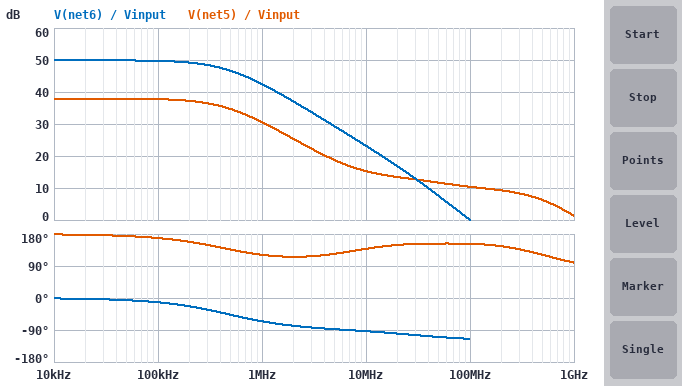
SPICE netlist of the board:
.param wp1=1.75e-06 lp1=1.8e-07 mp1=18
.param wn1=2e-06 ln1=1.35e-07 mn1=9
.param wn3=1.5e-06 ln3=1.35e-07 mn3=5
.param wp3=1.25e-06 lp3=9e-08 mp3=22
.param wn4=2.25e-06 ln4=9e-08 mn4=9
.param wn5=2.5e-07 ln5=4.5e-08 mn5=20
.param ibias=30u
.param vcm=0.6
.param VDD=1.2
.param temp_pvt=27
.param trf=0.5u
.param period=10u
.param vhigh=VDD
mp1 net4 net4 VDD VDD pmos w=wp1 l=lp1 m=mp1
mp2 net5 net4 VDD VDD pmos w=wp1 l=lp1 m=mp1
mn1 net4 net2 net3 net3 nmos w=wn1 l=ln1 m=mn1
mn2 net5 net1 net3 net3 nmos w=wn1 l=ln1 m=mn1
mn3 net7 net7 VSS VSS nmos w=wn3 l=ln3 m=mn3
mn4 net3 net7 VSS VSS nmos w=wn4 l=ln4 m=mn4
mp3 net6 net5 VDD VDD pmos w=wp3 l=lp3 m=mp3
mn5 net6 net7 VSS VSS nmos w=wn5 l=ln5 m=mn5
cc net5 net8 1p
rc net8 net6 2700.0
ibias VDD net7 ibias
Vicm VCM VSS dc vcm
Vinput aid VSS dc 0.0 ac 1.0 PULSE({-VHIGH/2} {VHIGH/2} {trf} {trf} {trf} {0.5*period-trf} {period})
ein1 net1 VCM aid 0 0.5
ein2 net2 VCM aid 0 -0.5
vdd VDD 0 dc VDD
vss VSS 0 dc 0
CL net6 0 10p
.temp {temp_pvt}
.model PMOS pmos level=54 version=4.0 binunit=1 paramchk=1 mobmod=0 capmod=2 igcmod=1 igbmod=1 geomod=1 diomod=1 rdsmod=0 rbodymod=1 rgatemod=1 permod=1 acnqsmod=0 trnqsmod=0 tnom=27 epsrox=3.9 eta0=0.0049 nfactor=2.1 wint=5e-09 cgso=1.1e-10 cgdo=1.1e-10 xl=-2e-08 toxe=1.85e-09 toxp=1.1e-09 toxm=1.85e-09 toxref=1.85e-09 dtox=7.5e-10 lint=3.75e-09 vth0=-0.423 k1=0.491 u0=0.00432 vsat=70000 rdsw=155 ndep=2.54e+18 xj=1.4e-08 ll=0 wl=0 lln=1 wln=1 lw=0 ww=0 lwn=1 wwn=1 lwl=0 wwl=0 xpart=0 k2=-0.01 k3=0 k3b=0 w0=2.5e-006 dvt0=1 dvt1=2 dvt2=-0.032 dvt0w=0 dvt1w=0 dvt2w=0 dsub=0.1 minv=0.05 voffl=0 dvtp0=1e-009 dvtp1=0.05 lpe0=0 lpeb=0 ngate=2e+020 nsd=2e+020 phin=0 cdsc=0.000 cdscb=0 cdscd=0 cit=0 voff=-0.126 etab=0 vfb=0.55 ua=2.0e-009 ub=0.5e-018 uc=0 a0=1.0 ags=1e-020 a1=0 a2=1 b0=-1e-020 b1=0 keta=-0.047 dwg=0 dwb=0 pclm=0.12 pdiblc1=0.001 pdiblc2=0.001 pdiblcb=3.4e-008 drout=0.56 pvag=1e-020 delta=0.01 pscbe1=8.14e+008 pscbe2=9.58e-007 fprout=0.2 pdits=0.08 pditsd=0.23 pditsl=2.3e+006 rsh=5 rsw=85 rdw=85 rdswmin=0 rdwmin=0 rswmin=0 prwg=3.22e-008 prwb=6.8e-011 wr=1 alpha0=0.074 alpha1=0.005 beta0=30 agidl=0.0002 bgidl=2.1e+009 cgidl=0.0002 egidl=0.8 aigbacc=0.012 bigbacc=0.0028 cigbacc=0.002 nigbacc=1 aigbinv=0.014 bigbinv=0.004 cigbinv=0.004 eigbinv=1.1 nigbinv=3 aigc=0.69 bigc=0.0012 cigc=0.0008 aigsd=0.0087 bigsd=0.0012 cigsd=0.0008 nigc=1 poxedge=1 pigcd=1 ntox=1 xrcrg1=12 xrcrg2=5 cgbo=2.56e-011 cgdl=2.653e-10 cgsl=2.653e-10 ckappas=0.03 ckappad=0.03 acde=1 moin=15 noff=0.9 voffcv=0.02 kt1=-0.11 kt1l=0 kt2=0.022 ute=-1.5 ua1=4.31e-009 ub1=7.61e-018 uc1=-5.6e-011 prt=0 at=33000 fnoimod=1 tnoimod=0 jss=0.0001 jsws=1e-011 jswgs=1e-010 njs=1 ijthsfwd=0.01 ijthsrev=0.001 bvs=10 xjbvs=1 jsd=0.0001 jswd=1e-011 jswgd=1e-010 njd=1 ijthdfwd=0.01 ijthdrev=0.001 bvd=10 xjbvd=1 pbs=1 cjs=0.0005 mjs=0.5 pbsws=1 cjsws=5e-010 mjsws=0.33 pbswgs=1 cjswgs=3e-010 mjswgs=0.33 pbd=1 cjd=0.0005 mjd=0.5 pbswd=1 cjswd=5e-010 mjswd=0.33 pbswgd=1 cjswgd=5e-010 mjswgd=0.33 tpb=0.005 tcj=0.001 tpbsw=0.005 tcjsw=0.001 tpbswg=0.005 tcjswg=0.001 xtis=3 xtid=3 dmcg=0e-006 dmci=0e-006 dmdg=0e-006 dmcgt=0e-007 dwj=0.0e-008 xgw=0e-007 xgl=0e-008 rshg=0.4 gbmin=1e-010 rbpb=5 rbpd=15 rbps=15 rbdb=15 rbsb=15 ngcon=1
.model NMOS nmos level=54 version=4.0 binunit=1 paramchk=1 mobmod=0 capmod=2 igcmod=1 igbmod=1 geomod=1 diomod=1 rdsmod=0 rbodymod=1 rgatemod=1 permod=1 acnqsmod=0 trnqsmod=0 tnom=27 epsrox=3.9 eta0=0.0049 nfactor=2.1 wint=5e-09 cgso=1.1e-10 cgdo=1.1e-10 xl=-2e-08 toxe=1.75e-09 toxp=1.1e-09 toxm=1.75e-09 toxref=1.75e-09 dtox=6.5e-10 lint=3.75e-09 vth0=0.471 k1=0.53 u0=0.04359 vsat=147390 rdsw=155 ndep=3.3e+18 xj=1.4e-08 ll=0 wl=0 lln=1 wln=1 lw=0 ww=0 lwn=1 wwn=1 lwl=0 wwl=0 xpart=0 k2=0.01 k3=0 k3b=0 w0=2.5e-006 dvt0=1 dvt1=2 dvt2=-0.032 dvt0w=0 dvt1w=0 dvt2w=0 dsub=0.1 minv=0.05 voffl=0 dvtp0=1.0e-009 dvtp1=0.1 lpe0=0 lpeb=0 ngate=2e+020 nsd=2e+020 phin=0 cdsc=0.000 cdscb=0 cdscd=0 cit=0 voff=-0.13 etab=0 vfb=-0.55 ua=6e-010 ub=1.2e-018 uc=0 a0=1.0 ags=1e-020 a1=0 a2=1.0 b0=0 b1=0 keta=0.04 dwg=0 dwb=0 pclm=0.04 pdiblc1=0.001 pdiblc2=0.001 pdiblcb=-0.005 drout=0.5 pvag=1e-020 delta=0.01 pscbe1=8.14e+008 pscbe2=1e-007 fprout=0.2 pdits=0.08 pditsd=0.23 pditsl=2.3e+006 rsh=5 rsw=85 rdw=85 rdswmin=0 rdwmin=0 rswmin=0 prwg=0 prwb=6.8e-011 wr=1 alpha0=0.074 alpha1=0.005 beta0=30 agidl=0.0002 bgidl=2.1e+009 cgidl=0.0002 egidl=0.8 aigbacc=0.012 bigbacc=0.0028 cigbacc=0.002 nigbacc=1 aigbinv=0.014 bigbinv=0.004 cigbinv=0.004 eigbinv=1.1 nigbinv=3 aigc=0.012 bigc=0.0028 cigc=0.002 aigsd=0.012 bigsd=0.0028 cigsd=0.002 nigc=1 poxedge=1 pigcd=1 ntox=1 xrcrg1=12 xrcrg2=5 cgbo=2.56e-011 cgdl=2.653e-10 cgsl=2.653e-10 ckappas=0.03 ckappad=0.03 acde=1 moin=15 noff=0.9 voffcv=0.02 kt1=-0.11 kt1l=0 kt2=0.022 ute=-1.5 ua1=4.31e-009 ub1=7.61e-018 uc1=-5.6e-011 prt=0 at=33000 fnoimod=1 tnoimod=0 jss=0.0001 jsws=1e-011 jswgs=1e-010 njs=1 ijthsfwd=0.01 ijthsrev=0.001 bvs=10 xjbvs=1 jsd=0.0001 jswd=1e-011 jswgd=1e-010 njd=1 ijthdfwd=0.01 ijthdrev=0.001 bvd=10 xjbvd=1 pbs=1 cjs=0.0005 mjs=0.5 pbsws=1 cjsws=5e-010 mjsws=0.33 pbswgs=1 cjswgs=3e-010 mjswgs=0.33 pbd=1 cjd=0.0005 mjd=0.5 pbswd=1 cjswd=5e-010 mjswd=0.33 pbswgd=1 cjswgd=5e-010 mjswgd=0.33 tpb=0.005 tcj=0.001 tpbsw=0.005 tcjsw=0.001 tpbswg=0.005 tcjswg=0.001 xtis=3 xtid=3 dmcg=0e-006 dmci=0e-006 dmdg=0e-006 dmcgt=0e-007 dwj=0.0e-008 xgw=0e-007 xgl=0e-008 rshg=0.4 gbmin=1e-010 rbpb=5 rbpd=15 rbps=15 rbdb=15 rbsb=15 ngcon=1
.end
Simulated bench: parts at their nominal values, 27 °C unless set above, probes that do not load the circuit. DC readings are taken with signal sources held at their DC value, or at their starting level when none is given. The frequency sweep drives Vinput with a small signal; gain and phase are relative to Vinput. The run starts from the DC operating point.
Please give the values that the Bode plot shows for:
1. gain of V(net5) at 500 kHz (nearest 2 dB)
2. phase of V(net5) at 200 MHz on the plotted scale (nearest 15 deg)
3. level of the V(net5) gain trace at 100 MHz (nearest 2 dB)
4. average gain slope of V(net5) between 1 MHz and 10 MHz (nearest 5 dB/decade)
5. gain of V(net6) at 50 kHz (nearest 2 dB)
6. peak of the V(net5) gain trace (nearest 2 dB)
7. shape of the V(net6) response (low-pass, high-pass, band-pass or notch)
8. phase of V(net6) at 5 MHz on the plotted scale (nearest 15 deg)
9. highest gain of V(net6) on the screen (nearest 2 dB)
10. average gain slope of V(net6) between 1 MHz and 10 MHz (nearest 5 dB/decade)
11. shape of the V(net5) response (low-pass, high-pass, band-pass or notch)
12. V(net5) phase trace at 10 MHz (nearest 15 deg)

34 dB
150 deg
10 dB
-15 dB/decade
50 dB
38 dB
low-pass
-90 deg
50 dB
-20 dB/decade
low-pass
135 deg
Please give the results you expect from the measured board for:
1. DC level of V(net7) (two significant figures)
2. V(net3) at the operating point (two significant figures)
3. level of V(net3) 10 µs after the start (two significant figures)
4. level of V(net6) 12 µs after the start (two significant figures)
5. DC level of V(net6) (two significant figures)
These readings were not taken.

430 mV
170 mV
430 mV
1.1 V
210 mV
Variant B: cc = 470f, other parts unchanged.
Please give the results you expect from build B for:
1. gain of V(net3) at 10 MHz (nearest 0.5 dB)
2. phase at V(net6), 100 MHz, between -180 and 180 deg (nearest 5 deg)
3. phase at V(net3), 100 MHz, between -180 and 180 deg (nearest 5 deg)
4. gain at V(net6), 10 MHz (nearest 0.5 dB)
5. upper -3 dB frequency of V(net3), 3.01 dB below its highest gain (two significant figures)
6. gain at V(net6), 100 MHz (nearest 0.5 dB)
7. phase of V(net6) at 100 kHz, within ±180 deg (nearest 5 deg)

-27.0 dB
-135 deg
150 deg
29.0 dB
940 kHz
2.5 dB
-5 deg
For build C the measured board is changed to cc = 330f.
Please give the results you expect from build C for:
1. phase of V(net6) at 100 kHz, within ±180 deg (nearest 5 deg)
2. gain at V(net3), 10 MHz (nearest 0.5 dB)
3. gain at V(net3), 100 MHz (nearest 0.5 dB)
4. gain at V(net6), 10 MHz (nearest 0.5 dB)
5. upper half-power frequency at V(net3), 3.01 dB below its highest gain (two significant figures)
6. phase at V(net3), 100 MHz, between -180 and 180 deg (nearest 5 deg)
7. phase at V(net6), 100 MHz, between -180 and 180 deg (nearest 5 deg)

-5 deg
-24.5 dB
-33.0 dB
31.5 dB
1.3 MHz
140 deg
-145 deg
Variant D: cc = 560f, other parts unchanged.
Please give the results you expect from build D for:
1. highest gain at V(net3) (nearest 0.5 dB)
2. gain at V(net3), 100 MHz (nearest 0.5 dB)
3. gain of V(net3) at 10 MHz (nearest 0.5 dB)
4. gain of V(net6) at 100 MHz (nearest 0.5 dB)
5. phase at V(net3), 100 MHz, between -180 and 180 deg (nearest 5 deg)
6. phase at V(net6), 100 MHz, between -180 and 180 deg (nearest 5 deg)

-10.5 dB
-35.5 dB
-28.5 dB
2.0 dB
155 deg
-130 deg
